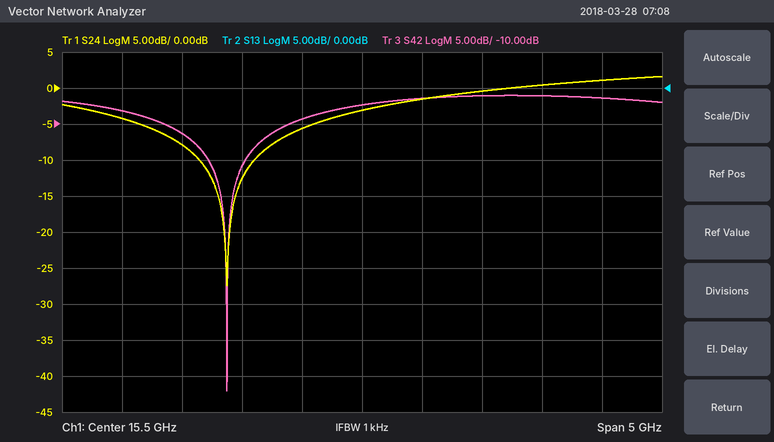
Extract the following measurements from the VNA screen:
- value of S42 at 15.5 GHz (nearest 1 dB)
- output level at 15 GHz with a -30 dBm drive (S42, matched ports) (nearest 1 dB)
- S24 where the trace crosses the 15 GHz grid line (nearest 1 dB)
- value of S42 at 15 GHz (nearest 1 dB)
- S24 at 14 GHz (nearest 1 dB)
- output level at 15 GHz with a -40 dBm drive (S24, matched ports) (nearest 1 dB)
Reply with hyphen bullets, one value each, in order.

- -7 dB
- -39 dBm
- -6 dB
- -9 dB
- -8 dB
- -46 dBm
